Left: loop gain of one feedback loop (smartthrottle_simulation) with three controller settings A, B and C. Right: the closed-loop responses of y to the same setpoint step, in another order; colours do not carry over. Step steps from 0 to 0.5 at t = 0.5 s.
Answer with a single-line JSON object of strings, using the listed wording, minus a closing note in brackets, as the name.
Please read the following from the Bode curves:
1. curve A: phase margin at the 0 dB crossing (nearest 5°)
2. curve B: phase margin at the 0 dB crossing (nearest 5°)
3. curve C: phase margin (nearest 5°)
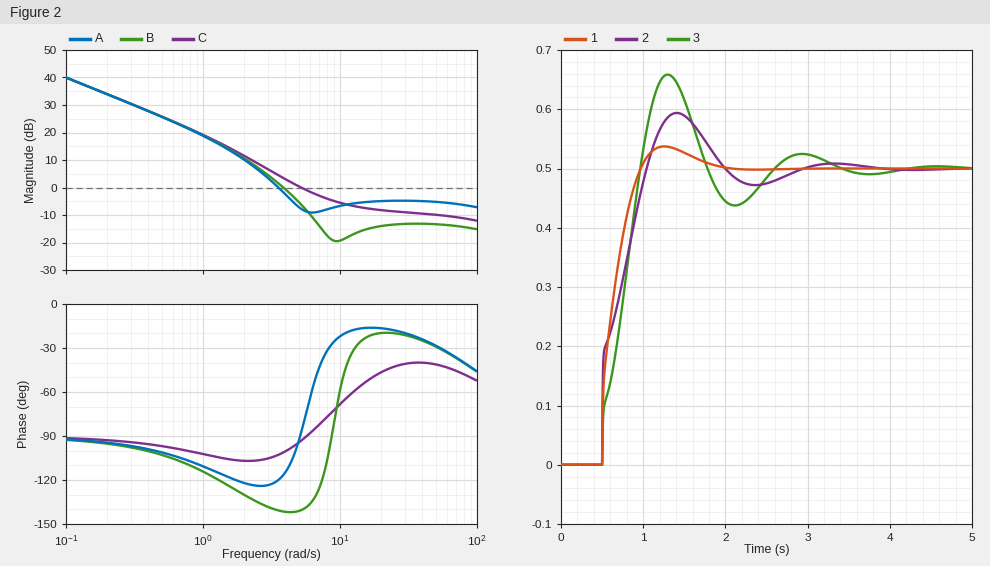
{"curve A: phase margin at the 0 dB crossing": "60°", "curve B: phase margin at the 0 dB crossing": "40°", "curve C: phase margin": "85°"}
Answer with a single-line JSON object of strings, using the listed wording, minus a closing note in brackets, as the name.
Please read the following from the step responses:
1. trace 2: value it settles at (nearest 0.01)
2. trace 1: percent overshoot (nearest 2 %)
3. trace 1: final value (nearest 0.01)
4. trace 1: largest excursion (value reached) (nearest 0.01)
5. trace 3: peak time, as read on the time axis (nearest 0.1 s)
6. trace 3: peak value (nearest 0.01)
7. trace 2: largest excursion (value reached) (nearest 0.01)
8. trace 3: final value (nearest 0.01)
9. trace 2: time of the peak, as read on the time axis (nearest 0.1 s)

{"trace 2: value it settles at": "0.50", "trace 1: percent overshoot": "8 %", "trace 1: final value": "0.50", "trace 1: largest excursion (value reached)": "0.54", "trace 3: peak time, as read on the time axis": "1.3 s", "trace 3: peak value": "0.66", "trace 2: largest excursion (value reached)": "0.59", "trace 3: final value": "0.50", "trace 2: time of the peak, as read on the time axis": "1.4 s"}
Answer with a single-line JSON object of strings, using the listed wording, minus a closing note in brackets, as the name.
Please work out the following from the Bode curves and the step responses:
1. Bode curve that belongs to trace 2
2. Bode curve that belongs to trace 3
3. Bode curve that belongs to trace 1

{"Bode curve that belongs to trace 2": "A", "Bode curve that belongs to trace 3": "B", "Bode curve that belongs to trace 1": "C"}
